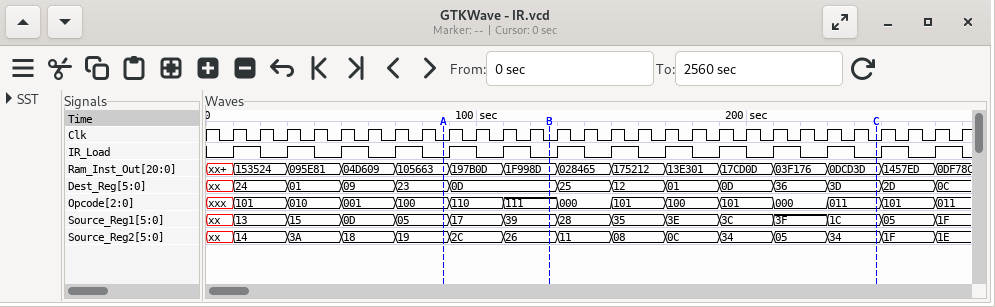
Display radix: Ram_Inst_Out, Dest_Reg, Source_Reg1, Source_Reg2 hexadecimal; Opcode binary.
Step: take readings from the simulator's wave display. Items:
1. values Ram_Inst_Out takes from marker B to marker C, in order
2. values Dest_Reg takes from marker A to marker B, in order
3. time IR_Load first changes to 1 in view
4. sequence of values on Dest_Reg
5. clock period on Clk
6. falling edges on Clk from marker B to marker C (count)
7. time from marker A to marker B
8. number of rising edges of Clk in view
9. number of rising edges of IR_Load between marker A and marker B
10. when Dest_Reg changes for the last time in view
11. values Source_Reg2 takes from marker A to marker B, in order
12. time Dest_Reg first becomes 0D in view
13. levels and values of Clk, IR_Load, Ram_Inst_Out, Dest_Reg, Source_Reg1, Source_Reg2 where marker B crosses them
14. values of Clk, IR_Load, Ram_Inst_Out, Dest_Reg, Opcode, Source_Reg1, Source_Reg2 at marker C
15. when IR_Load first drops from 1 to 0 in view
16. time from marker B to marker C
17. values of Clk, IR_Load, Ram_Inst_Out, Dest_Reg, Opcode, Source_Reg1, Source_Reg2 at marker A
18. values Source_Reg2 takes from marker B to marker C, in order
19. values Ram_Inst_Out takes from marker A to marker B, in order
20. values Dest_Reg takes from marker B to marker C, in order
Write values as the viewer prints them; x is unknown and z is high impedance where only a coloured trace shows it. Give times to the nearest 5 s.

1F998D, 028465, 175212, 13E301, 17CD0D, 03F176, 0DCD3D
23, 0D
10 s
xx, 24, 01, 09, 23, 0D, 25, 12, 01, 0D, 36, 3D, 2D, 0C
10 s
12
40 s
28
2
270 s
19, 2C, 26
90 s
Clk=0, IR_Load=0, Ram_Inst_Out=1F998D, Dest_Reg=0D, Source_Reg1=39, Source_Reg2=26
Clk=0, IR_Load=0, Ram_Inst_Out=0DCD3D, Dest_Reg=3D, Opcode=011, Source_Reg1=1C, Source_Reg2=34
20 s
120 s
Clk=0, IR_Load=0, Ram_Inst_Out=105663, Dest_Reg=23, Opcode=100, Source_Reg1=05, Source_Reg2=19
26, 11, 08, 0C, 34, 05, 34
105663, 197B0D, 1F998D
0D, 25, 12, 01, 0D, 36, 3D
